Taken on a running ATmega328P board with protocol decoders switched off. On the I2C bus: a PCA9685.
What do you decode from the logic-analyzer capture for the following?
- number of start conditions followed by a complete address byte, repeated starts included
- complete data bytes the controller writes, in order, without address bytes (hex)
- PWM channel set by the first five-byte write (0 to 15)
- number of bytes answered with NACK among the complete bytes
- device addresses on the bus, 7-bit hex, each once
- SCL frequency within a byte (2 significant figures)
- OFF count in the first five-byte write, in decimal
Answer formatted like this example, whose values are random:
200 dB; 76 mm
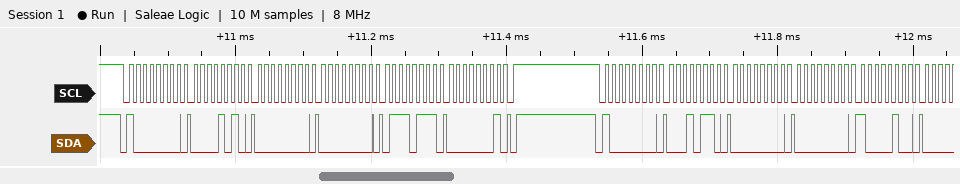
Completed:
2; 0A 00 00 77 01 16 00 00 84; 1; 0; 0x40; 100 kHz; 375
